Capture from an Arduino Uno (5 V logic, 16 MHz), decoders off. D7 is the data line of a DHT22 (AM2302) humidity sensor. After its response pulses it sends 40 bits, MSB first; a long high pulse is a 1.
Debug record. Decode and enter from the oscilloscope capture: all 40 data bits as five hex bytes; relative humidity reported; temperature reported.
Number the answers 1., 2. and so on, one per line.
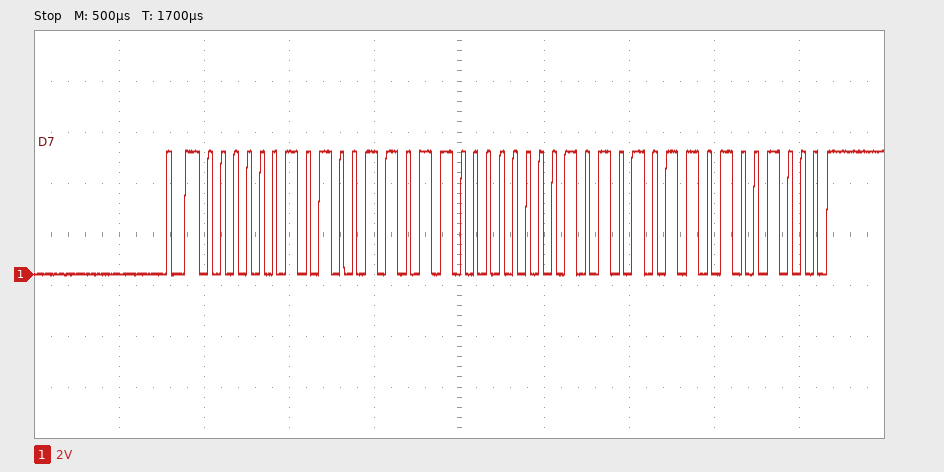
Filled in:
1. 02 9B 00 AB 48
2. 66.7 %
3. 17.1 °C
